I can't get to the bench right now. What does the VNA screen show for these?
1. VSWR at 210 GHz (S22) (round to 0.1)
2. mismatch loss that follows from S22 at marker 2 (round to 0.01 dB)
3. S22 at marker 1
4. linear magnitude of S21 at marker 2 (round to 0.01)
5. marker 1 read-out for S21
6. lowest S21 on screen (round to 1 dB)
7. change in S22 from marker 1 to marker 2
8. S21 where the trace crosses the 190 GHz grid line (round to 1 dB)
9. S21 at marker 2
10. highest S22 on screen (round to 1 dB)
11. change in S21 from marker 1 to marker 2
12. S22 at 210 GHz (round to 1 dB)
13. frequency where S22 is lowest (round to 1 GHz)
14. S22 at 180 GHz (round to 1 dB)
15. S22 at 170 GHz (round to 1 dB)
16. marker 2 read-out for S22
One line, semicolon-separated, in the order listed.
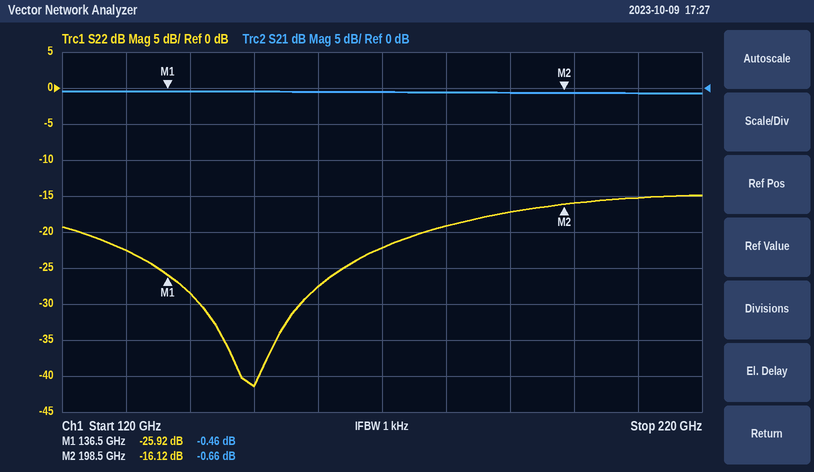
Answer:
1.4; 0.11 dB; -25.92 dB; 0.93; -0.46 dB; -1 dB; 9.80 dB; -1 dB; -0.66 dB; -15 dB; -0.20 dB; -15 dB; 150 GHz; -19 dB; -22 dB; -16.12 dB
